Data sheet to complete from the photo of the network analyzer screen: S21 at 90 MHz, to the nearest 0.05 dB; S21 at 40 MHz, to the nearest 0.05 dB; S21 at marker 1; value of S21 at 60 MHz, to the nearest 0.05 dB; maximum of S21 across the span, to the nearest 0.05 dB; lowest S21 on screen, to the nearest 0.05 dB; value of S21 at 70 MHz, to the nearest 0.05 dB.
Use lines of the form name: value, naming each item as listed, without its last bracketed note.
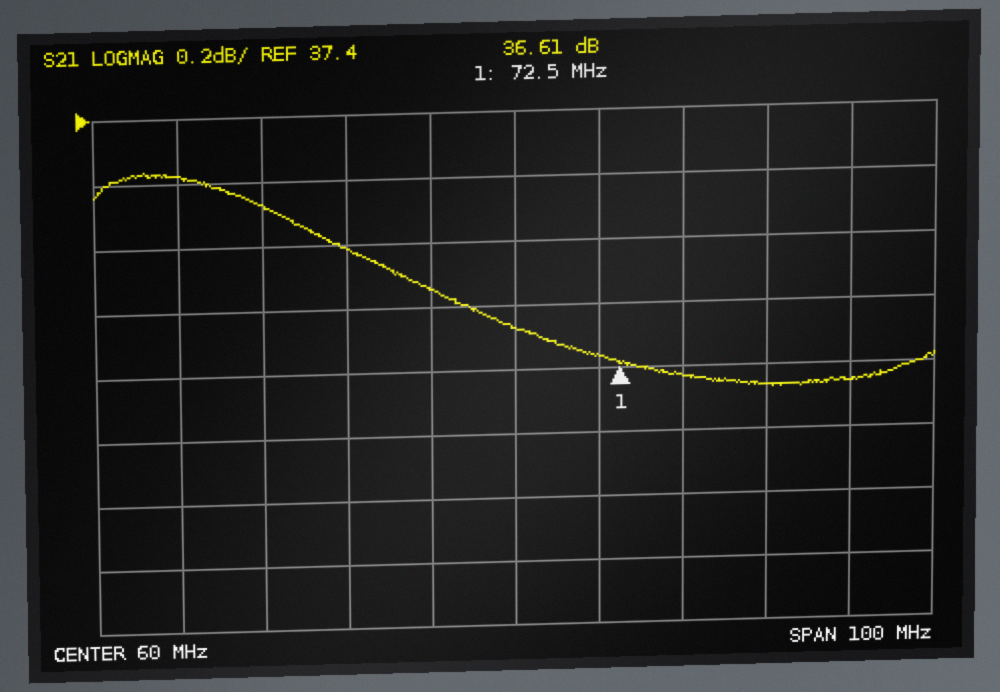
S21 at 90 MHz, to the nearest 0.05 dB: 36.55 dB
S21 at 40 MHz, to the nearest 0.05 dB: 37.00 dB
S21 at marker 1: 36.61 dB
value of S21 at 60 MHz, to the nearest 0.05 dB: 36.75 dB
maximum of S21 across the span, to the nearest 0.05 dB: 37.25 dB
lowest S21 on screen, to the nearest 0.05 dB: 36.55 dB
value of S21 at 70 MHz, to the nearest 0.05 dB: 36.65 dB
